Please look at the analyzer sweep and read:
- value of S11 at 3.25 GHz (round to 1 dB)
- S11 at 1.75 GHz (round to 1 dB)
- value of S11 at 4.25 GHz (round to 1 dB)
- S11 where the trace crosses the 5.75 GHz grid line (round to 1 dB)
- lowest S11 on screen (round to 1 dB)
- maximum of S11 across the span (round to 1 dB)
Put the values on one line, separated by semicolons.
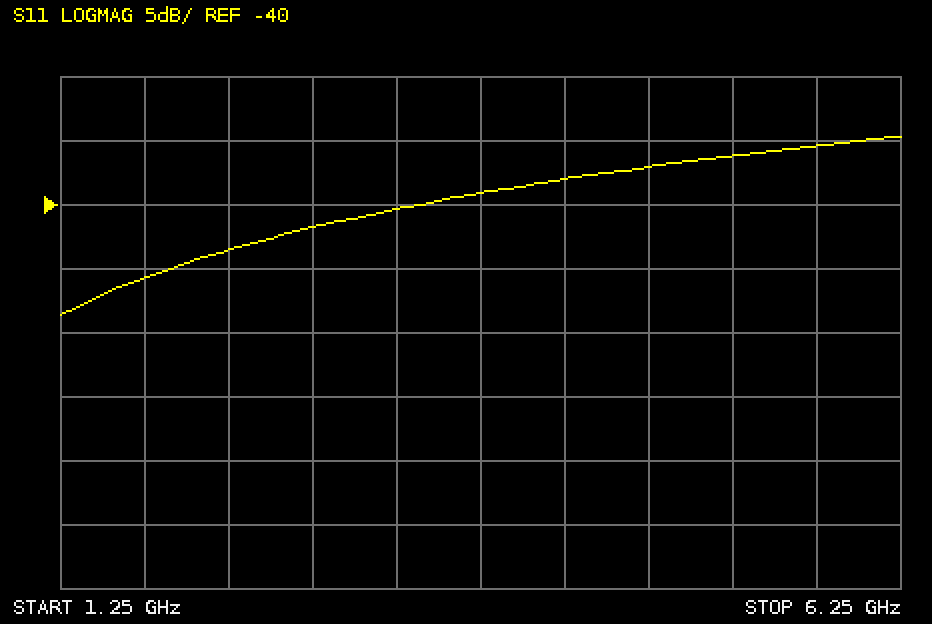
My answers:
-40 dB; -46 dB; -38 dB; -35 dB; -49 dB; -35 dB
